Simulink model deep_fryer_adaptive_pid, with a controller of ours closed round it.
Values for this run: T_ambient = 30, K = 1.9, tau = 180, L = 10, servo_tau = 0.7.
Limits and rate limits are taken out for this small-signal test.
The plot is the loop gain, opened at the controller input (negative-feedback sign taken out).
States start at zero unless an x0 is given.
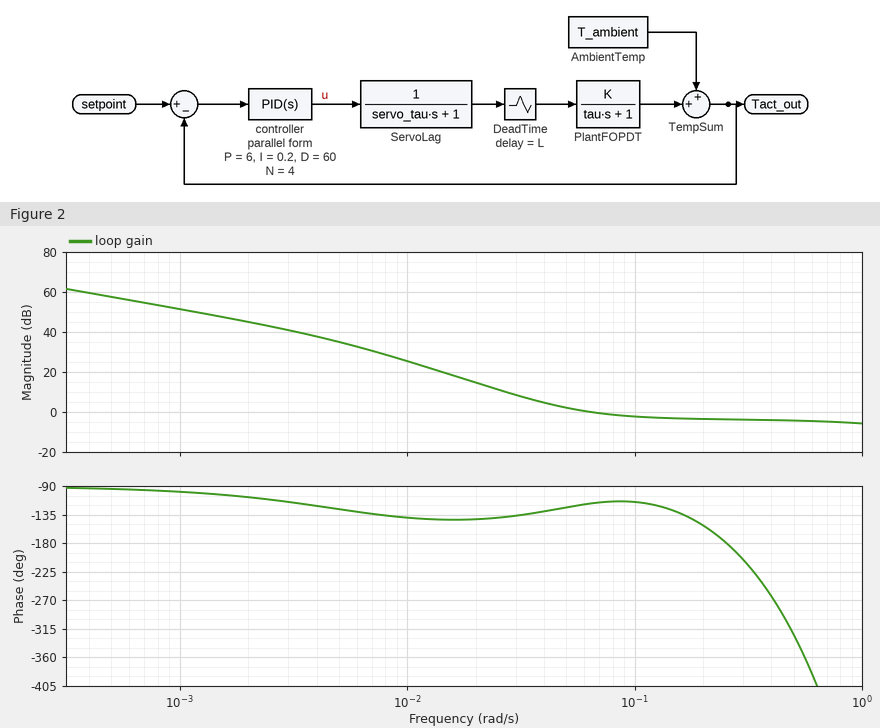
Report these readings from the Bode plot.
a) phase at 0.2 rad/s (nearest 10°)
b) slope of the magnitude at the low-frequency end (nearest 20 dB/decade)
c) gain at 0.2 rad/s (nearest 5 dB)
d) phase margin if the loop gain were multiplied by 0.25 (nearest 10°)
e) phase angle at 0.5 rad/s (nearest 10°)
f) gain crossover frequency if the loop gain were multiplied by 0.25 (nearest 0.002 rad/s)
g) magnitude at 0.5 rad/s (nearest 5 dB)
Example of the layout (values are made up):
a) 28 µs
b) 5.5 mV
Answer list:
a) -150°
b) -20 dB/decade
c) -5 dB
d) 40°
e) -320°
f) 0.024 rad/s
g) -5 dB
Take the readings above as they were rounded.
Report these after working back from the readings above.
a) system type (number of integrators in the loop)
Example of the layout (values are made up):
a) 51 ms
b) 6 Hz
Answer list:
a) 1
